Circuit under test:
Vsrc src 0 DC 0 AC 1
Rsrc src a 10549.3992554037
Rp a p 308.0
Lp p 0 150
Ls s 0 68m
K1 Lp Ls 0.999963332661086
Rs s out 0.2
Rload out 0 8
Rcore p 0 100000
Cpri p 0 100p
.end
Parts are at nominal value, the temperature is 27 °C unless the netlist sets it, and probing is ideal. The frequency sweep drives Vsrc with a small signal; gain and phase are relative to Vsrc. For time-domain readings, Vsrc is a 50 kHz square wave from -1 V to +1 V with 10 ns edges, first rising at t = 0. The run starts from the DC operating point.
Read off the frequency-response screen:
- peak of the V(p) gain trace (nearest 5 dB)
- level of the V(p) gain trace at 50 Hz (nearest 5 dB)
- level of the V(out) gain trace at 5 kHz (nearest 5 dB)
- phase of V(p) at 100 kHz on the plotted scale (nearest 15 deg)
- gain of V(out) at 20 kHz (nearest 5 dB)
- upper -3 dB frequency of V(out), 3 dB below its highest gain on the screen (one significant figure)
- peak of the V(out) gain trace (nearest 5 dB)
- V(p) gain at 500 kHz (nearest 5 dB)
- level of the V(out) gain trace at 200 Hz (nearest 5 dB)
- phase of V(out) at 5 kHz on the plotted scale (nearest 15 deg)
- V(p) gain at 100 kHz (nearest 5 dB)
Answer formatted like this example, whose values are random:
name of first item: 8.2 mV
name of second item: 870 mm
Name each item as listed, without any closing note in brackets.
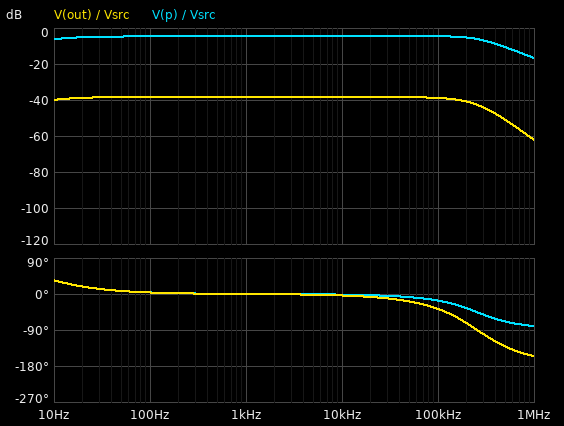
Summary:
peak of the V(p) gain trace: -5 dB
level of the V(p) gain trace at 50 Hz: -5 dB
level of the V(out) gain trace at 5 kHz: -40 dB
phase of V(p) at 100 kHz on the plotted scale: -15 deg
gain of V(out) at 20 kHz: -40 dB
upper -3 dB frequency of V(out), 3 dB below its highest gain on the screen: 200 kHz
peak of the V(out) gain trace: -40 dB
V(p) gain at 500 kHz: -10 dB
level of the V(out) gain trace at 200 Hz: -40 dB
phase of V(out) at 5 kHz on the plotted scale: 0 deg
V(p) gain at 100 kHz: -5 dB
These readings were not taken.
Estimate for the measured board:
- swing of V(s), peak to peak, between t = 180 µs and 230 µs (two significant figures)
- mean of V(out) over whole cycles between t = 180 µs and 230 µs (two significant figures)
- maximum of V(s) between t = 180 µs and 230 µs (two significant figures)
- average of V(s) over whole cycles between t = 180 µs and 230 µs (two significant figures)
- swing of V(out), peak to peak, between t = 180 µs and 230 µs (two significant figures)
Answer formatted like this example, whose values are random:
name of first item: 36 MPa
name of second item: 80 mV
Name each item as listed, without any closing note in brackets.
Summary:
swing of V(s), peak to peak, between t = 180 µs and 230 µs: 25 mV
mean of V(out) over whole cycles between t = 180 µs and 230 µs: 12 mV
maximum of V(s) between t = 180 µs and 230 µs: 25 mV
average of V(s) over whole cycles between t = 180 µs and 230 µs: 12 mV
swing of V(out), peak to peak, between t = 180 µs and 230 µs: 25 mV
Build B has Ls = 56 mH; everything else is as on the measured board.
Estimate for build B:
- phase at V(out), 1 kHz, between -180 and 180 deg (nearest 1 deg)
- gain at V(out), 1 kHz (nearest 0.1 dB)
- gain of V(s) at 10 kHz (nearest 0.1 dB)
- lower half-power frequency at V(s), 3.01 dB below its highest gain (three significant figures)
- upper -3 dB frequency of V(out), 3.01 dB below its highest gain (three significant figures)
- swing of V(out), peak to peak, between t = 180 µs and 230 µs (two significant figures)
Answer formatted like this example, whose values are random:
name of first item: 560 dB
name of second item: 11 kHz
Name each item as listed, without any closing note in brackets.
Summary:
phase at V(out), 1 kHz, between -180 and 180 deg: 0 deg
gain at V(out), 1 kHz: -38.6 dB
gain of V(s) at 10 kHz: -38.4 dB
lower half-power frequency at V(s), 3.01 dB below its highest gain: 7.19 Hz
upper -3 dB frequency of V(out), 3.01 dB below its highest gain: 211 kHz
swing of V(out), peak to peak, between t = 180 µs and 230 µs: 24 mV
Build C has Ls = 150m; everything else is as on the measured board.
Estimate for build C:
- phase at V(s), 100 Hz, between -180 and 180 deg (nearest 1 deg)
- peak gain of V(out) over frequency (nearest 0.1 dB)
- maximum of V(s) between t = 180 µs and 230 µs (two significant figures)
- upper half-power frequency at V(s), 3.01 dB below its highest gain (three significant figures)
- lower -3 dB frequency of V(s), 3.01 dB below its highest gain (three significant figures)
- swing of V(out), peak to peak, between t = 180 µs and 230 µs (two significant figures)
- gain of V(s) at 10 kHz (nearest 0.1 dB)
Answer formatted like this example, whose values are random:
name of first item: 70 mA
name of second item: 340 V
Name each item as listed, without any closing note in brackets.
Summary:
phase at V(s), 100 Hz, between -180 and 180 deg: 3 deg
peak gain of V(out) over frequency: -37.9 dB
maximum of V(s) between t = 180 µs and 230 µs: 27 mV
upper half-power frequency at V(s), 3.01 dB below its highest gain: 212 kHz
lower -3 dB frequency of V(s), 3.01 dB below its highest gain: 4.76 Hz
swing of V(out), peak to peak, between t = 180 µs and 230 µs: 28 mV
gain of V(s) at 10 kHz: -37.7 dB
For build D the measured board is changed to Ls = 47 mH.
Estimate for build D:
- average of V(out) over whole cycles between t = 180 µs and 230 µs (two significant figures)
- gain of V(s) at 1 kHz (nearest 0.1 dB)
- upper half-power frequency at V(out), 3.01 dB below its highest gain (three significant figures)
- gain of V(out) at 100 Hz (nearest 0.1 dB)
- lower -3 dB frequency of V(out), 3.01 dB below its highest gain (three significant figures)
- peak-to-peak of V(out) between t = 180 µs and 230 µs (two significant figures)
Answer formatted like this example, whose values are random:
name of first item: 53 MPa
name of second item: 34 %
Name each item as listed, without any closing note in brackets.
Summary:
average of V(out) over whole cycles between t = 180 µs and 230 µs: 11 mV
gain of V(s) at 1 kHz: -38.7 dB
upper half-power frequency at V(out), 3.01 dB below its highest gain: 207 kHz
gain of V(out) at 100 Hz: -38.9 dB
lower -3 dB frequency of V(out), 3.01 dB below its highest gain: 7.56 Hz
peak-to-peak of V(out) between t = 180 µs and 230 µs: 23 mV
